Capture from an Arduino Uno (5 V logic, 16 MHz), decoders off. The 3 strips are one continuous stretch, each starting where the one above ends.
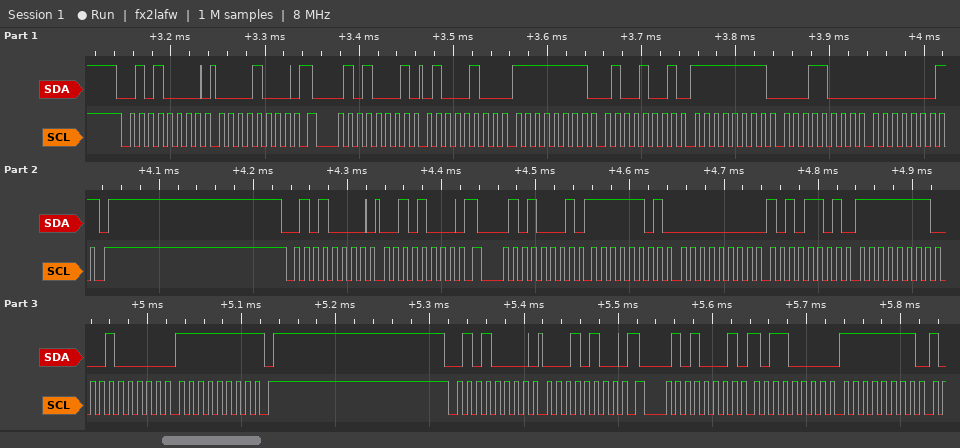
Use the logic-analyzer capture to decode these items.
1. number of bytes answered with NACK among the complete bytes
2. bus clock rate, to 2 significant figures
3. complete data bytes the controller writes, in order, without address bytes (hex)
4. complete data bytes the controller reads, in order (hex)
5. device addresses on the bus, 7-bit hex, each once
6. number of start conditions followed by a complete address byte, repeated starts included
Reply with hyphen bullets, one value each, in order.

- 2
- 100 kHz
- 08 28 14
- 44 FF 49 FF 18 01 FD 00 AD FF 20 FF B0 FF
- 0x28
- 6
